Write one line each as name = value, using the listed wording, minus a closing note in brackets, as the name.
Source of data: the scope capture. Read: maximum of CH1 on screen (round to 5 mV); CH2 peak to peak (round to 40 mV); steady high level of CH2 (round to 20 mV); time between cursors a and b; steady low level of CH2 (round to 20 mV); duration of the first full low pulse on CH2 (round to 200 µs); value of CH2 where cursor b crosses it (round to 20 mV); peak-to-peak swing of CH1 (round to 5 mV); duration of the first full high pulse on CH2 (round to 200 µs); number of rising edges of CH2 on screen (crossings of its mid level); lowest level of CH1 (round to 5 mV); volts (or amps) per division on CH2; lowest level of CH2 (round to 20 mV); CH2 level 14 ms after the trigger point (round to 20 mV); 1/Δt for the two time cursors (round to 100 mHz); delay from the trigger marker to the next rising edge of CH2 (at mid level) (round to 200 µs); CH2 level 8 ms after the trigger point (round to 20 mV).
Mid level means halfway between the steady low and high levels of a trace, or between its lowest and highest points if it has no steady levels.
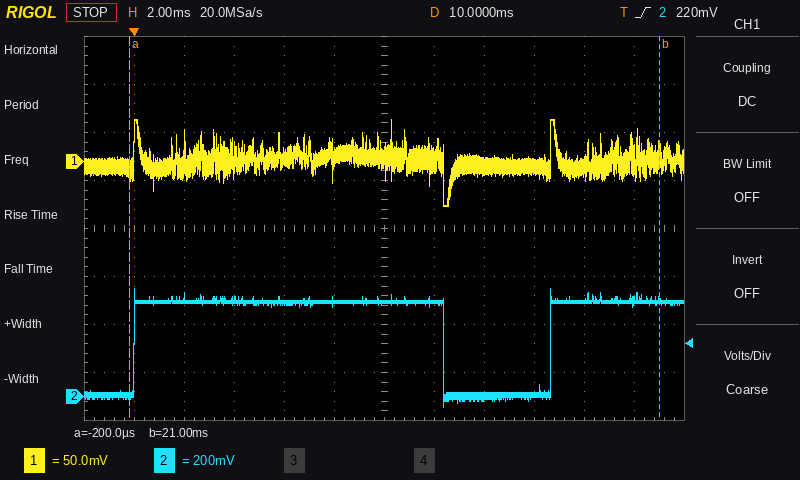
maximum of CH1 on screen = 45 mV
CH2 peak to peak = 480 mV
steady high level of CH2 = 400 mV
time between cursors a and b = 21.2 ms
steady low level of CH2 = 0 mV
duration of the first full low pulse on CH2 = 4.2 ms
value of CH2 where cursor b crosses it = 400 mV
peak-to-peak swing of CH1 = 90 mV
duration of the first full high pulse on CH2 = 12.4 ms
number of rising edges of CH2 on screen = 2
lowest level of CH1 = -45 mV
volts (or amps) per division on CH2 = 200 mV
lowest level of CH2 = -40 mV
CH2 level 14 ms after the trigger point = 0 mV
1/Δt for the two time cursors = 47.2 Hz
delay from the trigger marker to the next rising edge of CH2 (at mid level) = 16.6 ms
CH2 level 8 ms after the trigger point = 400 mV
